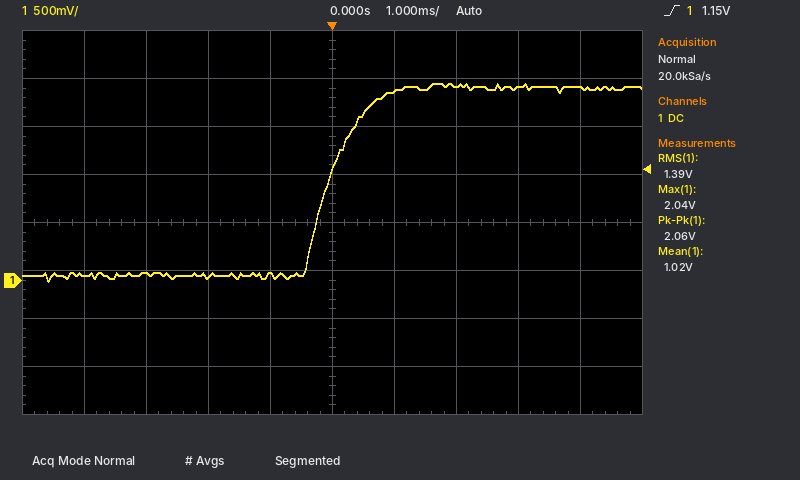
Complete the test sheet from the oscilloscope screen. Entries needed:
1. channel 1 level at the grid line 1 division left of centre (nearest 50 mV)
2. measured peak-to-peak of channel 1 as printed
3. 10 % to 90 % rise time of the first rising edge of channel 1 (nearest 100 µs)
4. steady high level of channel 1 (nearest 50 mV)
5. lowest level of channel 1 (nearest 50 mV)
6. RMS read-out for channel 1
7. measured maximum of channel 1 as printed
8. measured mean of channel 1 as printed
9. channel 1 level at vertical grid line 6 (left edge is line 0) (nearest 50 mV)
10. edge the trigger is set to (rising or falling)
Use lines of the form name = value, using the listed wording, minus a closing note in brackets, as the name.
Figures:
channel 1 level at the grid line 1 division left of centre = 50 mV
measured peak-to-peak of channel 1 as printed = 2.06 V
10 % to 90 % rise time of the first rising edge of channel 1 = 1.0 ms
steady high level of channel 1 = 2.00 V
lowest level of channel 1 = 0 mV
RMS read-out for channel 1 = 1.39 V
measured maximum of channel 1 as printed = 2.04 V
measured mean of channel 1 as printed = 1.02 V
channel 1 level at vertical grid line 6 (left edge is line 0) = 1.95 V
edge the trigger is set to = rising
